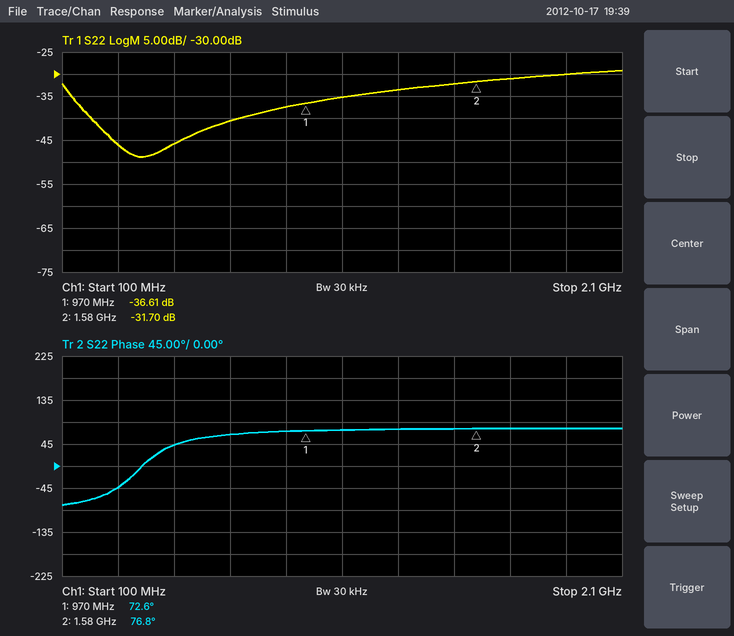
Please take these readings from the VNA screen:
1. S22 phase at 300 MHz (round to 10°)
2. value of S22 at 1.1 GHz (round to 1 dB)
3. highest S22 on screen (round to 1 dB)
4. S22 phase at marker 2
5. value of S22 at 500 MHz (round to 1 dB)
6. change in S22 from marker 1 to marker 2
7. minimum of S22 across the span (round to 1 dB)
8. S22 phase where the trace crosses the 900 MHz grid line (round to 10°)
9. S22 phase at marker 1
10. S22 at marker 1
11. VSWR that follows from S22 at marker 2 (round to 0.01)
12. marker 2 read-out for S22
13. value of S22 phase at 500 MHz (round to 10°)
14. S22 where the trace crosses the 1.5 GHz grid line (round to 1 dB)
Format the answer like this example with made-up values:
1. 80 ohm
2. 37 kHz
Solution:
1. -40°
2. -35 dB
3. -29 dB
4. 76.8°
5. -46 dB
6. 4.91 dB
7. -49 dB
8. 70°
9. 72.6°
10. -36.61 dB
11. 1.05
12. -31.70 dB
13. 40°
14. -32 dB
